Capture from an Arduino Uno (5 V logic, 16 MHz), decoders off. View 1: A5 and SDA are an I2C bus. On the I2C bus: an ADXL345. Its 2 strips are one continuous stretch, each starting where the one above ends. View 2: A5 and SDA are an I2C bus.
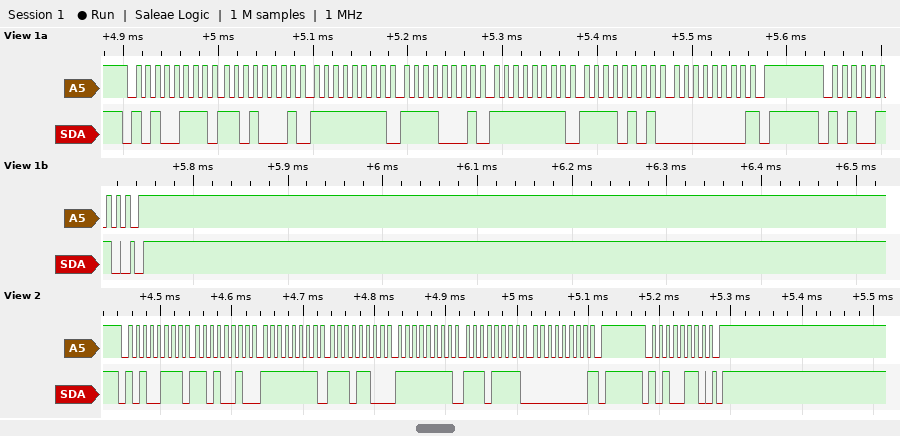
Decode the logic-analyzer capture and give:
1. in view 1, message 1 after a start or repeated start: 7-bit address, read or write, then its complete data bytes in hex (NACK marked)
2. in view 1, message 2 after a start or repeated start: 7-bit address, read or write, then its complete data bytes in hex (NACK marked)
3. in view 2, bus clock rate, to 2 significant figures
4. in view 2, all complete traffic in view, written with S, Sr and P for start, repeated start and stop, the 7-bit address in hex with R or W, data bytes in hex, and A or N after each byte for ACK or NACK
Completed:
0x53 read: D1 FF F1 FF F5 00 NACK
0x53 write
100 kHz
S 53R A D2 A FF A EC A FF A EF A 00 N P S 53W A P
